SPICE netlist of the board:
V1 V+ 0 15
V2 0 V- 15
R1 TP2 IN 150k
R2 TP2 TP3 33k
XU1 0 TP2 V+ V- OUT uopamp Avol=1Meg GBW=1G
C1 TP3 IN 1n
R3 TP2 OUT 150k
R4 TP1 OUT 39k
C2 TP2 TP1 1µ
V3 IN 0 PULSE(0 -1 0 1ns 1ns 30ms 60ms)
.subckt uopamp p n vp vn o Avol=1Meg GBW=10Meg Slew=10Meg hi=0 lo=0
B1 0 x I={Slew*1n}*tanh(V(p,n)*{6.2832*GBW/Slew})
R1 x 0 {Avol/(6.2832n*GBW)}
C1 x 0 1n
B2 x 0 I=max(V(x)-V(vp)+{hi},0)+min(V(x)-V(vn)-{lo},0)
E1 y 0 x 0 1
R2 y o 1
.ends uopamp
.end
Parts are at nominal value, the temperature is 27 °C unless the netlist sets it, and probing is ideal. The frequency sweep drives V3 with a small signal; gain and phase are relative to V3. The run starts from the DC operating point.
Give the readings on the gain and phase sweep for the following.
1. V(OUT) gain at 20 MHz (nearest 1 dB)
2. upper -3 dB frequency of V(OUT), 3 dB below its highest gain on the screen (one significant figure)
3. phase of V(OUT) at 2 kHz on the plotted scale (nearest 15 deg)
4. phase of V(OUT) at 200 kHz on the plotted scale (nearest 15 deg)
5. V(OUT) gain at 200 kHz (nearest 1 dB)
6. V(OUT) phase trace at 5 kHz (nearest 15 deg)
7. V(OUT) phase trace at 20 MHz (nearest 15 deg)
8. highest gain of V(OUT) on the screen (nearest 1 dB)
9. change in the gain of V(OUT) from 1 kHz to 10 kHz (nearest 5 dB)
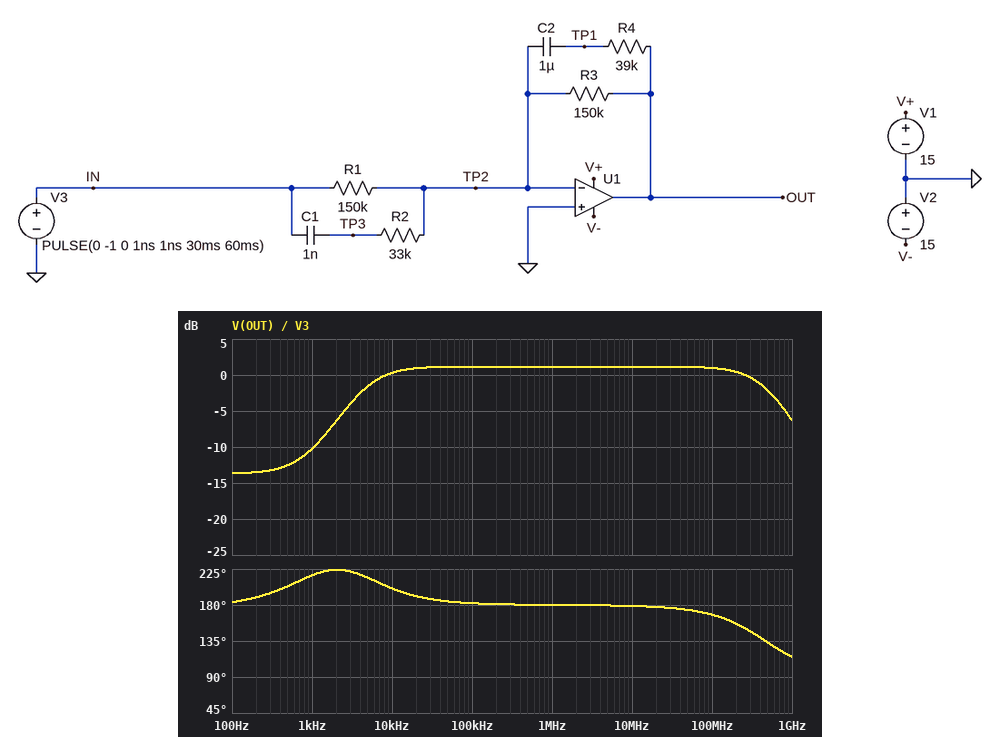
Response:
1 dB
500 MHz
225 deg
180 deg
1 dB
210 deg
180 deg
1 dB
10 dB
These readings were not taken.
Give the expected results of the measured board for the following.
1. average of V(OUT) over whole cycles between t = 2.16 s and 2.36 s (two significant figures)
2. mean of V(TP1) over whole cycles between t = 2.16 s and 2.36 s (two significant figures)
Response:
500 mV
500 mV
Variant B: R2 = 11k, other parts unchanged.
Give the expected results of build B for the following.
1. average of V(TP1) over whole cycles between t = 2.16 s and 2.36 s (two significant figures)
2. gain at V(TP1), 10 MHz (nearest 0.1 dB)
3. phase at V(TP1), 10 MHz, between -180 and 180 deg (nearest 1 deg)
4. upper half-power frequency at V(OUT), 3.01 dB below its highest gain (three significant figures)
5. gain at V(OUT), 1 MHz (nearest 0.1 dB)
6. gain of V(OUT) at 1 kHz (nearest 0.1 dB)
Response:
500 mV
-30.4 dB
88 deg
249 MHz
9.6 dB
-10.7 dB
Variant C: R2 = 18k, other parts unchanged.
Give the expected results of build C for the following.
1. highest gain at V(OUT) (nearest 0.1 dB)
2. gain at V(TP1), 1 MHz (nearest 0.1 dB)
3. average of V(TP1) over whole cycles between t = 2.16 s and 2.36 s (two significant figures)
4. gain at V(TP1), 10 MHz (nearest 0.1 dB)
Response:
5.7 dB
-54.3 dB
500 mV
-34.3 dB
